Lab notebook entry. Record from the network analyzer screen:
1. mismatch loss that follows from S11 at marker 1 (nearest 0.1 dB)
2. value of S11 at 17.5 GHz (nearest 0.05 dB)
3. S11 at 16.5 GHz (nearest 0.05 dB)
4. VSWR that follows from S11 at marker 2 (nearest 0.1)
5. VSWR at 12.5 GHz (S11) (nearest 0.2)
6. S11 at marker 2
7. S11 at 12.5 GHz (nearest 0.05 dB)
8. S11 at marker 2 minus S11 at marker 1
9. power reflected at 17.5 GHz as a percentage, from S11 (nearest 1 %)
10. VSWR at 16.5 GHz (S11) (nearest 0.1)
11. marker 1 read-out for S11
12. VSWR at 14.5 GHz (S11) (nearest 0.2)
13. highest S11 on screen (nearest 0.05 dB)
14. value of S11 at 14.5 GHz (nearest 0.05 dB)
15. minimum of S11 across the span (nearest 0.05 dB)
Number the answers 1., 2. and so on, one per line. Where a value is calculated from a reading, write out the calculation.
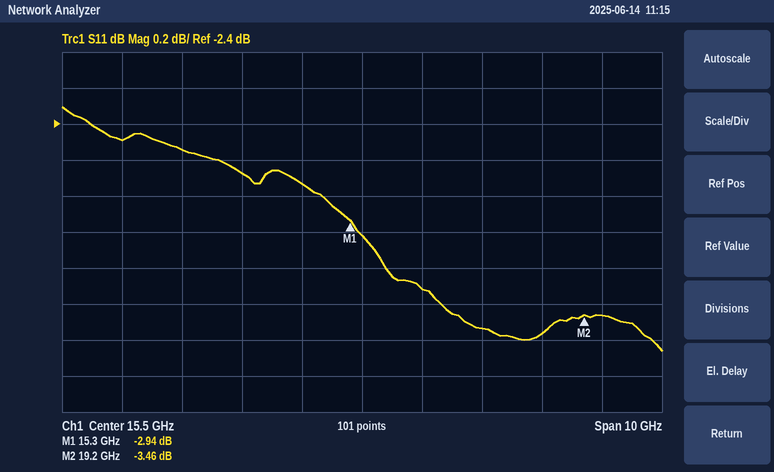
1. −10 log10(1 − 10^(-2.94/10)) ≈ 3.1 dB
2. -3.55 dB
3. -3.30 dB
4. (1 + 0.6714)/(1 − 0.6714) ≈ 5.1
5. |Γ| = 10^(-2.55/20) = 0.7456; VSWR = (1 + 0.7456)/(1 − 0.7456) ≈ 6.86, so 6.8 to the nearest 0.2
6. -3.46 dB
7. -2.55 dB
8. -3.46 − (-2.94) = -0.52 dB
9. 10^(-3.55/10) ≈ 44 %
10. |Γ| = 10^(-3.3/20) = 0.6839; VSWR = (1 + 0.6839)/(1 − 0.6839) ≈ 5.3
11. -2.94 dB
12. |Γ| = 10^(-2.75/20) = 0.7286; VSWR = (1 + 0.7286)/(1 − 0.7286) ≈ 6.4
13. -2.30 dB
14. -2.75 dB
15. -3.65 dB
